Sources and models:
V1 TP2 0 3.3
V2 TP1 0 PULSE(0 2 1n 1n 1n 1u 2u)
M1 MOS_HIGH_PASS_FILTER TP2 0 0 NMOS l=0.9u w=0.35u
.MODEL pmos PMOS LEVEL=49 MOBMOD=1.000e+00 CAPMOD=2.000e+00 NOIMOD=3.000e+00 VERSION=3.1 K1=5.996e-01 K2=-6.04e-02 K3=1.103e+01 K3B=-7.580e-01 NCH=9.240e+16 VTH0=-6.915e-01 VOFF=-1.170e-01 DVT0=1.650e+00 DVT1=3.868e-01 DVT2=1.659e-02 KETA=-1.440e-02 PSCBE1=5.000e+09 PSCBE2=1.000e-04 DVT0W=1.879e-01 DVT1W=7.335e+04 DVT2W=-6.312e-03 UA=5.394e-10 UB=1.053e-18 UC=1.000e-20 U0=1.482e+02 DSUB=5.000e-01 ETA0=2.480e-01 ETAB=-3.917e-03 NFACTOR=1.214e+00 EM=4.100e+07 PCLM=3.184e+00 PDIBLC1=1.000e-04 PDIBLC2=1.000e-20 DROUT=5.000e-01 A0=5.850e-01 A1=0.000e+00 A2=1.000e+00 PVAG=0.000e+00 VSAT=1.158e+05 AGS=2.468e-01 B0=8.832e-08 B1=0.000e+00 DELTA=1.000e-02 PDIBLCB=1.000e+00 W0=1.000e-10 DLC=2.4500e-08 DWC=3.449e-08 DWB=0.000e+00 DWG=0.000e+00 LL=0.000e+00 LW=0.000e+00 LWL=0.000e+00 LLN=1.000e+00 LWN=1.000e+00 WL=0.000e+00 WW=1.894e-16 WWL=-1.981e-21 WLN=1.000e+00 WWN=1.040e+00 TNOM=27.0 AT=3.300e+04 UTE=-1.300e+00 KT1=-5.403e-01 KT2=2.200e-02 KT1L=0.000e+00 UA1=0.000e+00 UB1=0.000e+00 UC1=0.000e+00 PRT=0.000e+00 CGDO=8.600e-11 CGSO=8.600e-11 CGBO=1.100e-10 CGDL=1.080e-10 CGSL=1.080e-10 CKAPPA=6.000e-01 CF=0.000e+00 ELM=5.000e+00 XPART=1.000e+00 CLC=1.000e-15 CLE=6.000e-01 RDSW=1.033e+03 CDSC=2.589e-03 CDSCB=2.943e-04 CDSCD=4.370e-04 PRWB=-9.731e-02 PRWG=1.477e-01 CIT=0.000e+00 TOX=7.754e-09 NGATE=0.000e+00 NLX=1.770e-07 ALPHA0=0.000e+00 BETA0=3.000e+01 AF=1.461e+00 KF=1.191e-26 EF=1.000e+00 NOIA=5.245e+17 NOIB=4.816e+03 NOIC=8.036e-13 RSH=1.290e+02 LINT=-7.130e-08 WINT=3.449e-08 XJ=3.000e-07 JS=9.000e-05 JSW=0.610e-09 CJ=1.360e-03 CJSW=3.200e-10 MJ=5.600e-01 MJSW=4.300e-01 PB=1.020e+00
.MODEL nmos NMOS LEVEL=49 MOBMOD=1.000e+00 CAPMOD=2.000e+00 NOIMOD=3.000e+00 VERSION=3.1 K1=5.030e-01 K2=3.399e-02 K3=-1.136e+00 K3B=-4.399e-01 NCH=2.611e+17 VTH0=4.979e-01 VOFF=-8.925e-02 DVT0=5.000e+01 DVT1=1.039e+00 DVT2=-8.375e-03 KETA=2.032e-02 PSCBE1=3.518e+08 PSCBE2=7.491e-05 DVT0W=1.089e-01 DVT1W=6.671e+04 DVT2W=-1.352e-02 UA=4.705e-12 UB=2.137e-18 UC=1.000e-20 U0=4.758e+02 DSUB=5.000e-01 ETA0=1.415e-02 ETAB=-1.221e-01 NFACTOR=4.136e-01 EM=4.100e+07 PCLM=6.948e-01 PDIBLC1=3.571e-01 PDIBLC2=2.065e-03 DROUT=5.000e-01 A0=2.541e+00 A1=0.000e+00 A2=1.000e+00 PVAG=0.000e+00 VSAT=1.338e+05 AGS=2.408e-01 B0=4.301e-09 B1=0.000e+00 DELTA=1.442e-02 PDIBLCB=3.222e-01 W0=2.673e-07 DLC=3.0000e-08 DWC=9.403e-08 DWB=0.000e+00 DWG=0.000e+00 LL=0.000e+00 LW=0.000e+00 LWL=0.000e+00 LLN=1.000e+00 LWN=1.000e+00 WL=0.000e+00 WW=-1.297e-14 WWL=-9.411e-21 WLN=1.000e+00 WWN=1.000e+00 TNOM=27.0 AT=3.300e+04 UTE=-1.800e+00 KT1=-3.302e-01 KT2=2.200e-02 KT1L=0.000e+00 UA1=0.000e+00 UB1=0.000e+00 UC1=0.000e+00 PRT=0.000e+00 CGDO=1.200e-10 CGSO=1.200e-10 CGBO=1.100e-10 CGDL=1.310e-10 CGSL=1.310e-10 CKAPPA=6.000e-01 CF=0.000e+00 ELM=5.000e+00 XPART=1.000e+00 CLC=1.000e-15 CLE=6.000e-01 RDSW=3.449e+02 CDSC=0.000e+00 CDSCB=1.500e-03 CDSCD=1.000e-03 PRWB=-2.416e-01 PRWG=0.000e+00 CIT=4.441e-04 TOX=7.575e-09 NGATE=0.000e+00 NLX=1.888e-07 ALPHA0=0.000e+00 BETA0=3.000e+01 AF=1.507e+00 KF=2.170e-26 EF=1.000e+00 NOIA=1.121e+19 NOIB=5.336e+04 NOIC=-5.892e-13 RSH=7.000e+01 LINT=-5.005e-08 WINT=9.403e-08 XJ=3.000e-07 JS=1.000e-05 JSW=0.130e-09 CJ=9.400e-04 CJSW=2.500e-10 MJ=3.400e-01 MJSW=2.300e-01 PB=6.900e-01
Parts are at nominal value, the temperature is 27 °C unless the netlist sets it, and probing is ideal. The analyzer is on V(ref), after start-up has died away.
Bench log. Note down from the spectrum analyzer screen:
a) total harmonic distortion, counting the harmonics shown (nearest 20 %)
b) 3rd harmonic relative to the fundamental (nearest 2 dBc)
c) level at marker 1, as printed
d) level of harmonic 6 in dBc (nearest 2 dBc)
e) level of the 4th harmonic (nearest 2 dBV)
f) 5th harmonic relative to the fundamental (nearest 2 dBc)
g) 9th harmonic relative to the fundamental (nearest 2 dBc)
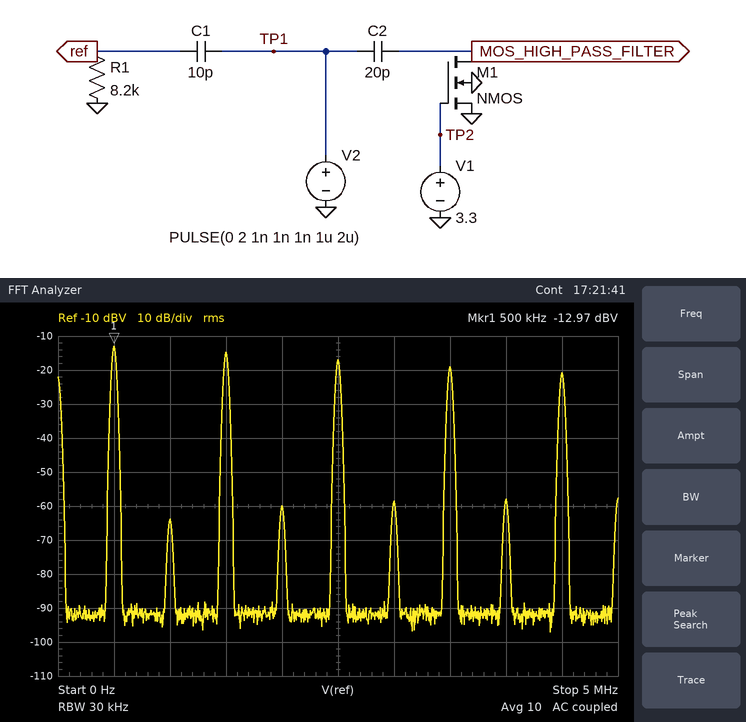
120 %
-2 dBc
-12.97 dBV
-46 dBc
-60 dBV
-4 dBc
-8 dBc
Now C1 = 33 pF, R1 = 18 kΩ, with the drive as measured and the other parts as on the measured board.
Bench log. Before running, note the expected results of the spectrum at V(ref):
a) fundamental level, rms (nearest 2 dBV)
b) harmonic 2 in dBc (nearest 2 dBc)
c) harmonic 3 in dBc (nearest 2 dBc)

-2 dBV
-56 dBc
-8 dBc
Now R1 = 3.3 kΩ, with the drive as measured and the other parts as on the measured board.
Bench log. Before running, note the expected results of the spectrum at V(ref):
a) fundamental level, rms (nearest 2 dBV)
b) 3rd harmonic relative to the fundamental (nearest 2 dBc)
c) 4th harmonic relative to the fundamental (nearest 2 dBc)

-20 dBV
0 dBc
-44 dBc
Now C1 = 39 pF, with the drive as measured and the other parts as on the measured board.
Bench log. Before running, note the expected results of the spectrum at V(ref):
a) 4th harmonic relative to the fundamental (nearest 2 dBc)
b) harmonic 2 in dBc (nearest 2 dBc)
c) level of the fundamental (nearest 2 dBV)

-54 dBc
-54 dBc
-4 dBV
